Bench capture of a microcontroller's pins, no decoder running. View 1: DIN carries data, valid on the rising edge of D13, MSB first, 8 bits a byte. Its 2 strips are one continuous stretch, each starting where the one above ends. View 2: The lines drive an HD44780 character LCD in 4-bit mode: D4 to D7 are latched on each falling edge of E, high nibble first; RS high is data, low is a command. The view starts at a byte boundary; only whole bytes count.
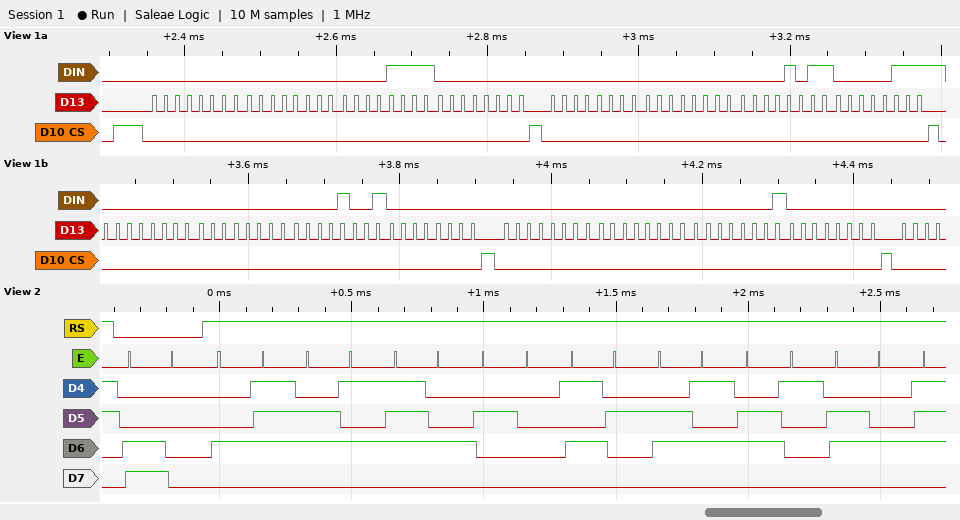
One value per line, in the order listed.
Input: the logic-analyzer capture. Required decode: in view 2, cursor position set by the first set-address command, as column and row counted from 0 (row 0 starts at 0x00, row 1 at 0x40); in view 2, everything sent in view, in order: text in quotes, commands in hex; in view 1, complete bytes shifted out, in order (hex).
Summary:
column 0, row 1
0xC0 "Get Read"
0x00 0x00 0x0F 0x00 0x00 0x00 0x0B 0x07 0x00 0x00 0x09 0x00 0x00 0x00 0x01 0x00
